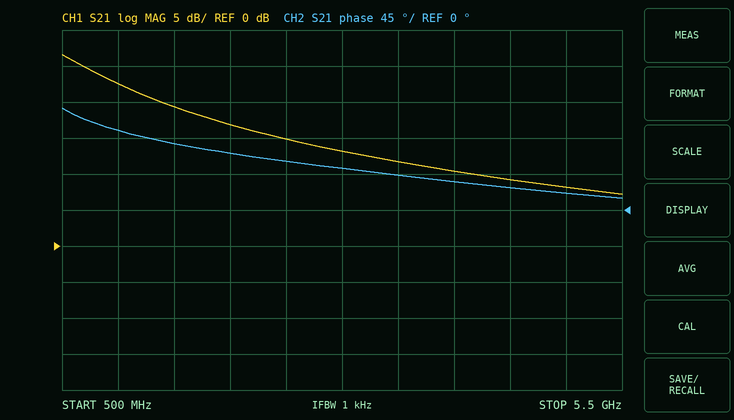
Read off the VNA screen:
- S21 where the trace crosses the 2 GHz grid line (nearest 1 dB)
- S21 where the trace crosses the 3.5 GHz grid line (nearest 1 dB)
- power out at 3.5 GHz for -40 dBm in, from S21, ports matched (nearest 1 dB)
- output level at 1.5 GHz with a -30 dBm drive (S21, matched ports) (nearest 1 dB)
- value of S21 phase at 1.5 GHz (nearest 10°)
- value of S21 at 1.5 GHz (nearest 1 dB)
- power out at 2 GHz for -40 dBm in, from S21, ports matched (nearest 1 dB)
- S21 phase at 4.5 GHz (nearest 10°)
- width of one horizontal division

17 dB
12 dB
-28 dBm
-11 dBm
80°
19 dB
-23 dBm
30°
500 MHz
